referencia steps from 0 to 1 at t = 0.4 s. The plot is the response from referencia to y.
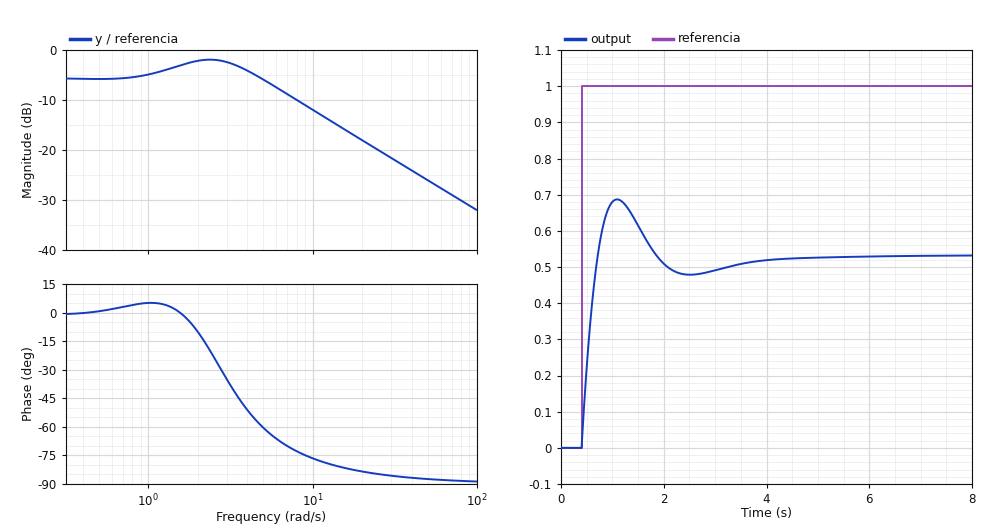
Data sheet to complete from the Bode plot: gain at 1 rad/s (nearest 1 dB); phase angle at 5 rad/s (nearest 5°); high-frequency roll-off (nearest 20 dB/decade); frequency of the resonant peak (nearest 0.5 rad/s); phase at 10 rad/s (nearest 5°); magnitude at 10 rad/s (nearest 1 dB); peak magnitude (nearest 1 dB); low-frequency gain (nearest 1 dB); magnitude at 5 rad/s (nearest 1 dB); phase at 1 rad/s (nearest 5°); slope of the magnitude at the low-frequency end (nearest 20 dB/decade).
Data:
-5 dB
-60°
-20 dB/decade
2.5 rad/s
-75°
-12 dB
-2 dB
-6 dB
-6 dB
5°
0 dB/decade
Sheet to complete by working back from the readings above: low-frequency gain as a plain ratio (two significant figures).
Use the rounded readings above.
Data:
0.50
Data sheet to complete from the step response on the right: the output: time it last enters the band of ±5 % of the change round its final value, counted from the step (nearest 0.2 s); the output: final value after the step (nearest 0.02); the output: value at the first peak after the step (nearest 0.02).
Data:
3.0 s
0.54
0.68
